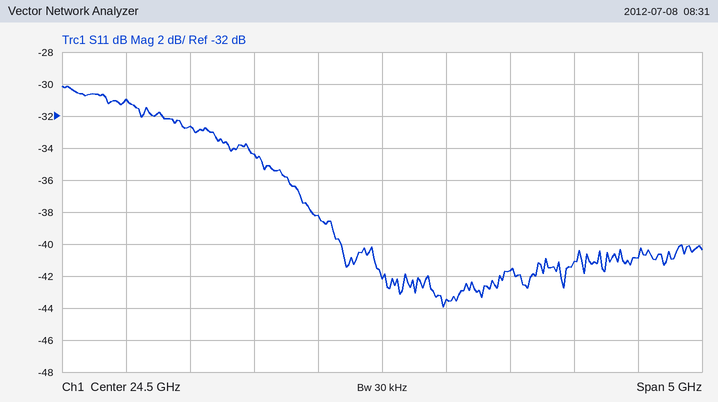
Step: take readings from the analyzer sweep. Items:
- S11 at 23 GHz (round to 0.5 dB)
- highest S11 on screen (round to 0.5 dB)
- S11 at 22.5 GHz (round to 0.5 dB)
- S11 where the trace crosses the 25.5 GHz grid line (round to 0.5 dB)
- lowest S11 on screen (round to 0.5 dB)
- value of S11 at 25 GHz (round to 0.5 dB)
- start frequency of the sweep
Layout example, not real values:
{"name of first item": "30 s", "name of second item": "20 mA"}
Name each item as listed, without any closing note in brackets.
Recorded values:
{"S11 at 23 GHz": "-32.5 dB", "highest S11 on screen": "-30.0 dB", "S11 at 22.5 GHz": "-31.0 dB", "S11 where the trace crosses the 25.5 GHz grid line": "-41.5 dB", "lowest S11 on screen": "-44.0 dB", "value of S11 at 25 GHz": "-43.5 dB", "start frequency of the sweep": "22 GHz"}
